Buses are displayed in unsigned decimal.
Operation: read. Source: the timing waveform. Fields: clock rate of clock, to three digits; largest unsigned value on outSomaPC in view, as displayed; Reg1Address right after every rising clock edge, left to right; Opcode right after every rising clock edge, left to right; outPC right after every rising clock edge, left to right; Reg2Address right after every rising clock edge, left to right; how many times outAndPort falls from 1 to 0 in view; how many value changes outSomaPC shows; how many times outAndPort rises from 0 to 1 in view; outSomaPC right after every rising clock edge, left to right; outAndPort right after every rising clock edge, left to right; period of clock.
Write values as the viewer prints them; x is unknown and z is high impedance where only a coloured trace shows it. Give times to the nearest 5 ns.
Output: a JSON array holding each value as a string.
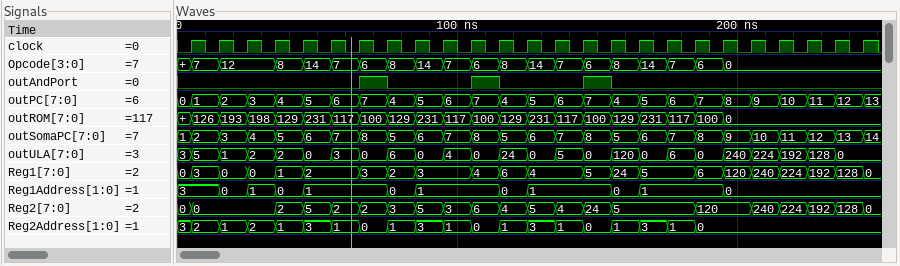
["100 MHz", "14", "3, 0, 1, 0, 1, 1, 1, 0, 1, 1, 1, 0, 1, 1, 1, 0, 1, 1, 1, 0, 0, 0, 0, 0, 0", "7, 12, 12, 8, 14, 7, 6, 8, 14, 7, 6, 8, 14, 7, 6, 8, 14, 7, 6, 0, 0, 0, 0, 0, 0", "1, 2, 3, 4, 5, 6, 7, 4, 5, 6, 7, 4, 5, 6, 7, 4, 5, 6, 7, 8, 9, 10, 11, 12, 13", "2, 1, 2, 1, 3, 1, 0, 1, 3, 1, 0, 1, 3, 1, 0, 1, 3, 1, 0, 0, 0, 0, 0, 0, 0", "3", "25", "3", "2, 3, 4, 5, 6, 7, 8, 5, 6, 7, 8, 5, 6, 7, 8, 5, 6, 7, 8, 9, 10, 11, 12, 13, 14", "0 0 0 0 0 0 1 0 0 0 1 0 0 0 1 0 0 0 0 0 0 0 0 0 0", "10 ns"]
